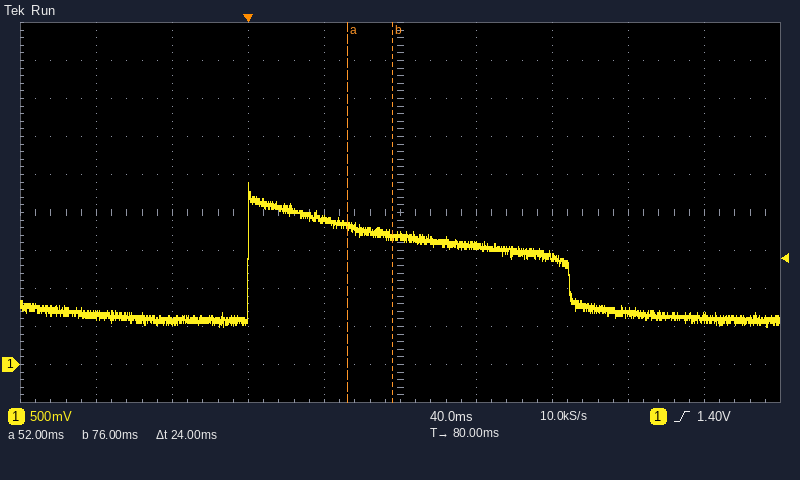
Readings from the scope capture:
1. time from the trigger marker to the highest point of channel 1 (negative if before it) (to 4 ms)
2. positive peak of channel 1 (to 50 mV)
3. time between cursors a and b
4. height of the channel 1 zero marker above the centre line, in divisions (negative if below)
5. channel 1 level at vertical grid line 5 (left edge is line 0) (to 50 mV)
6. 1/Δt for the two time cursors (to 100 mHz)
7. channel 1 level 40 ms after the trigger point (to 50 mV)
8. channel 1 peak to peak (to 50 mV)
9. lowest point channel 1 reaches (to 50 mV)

0 ms
2.40 V
24 ms
-4.0 div
1.70 V
41.7 Hz
1.90 V
1.90 V
500 mV
